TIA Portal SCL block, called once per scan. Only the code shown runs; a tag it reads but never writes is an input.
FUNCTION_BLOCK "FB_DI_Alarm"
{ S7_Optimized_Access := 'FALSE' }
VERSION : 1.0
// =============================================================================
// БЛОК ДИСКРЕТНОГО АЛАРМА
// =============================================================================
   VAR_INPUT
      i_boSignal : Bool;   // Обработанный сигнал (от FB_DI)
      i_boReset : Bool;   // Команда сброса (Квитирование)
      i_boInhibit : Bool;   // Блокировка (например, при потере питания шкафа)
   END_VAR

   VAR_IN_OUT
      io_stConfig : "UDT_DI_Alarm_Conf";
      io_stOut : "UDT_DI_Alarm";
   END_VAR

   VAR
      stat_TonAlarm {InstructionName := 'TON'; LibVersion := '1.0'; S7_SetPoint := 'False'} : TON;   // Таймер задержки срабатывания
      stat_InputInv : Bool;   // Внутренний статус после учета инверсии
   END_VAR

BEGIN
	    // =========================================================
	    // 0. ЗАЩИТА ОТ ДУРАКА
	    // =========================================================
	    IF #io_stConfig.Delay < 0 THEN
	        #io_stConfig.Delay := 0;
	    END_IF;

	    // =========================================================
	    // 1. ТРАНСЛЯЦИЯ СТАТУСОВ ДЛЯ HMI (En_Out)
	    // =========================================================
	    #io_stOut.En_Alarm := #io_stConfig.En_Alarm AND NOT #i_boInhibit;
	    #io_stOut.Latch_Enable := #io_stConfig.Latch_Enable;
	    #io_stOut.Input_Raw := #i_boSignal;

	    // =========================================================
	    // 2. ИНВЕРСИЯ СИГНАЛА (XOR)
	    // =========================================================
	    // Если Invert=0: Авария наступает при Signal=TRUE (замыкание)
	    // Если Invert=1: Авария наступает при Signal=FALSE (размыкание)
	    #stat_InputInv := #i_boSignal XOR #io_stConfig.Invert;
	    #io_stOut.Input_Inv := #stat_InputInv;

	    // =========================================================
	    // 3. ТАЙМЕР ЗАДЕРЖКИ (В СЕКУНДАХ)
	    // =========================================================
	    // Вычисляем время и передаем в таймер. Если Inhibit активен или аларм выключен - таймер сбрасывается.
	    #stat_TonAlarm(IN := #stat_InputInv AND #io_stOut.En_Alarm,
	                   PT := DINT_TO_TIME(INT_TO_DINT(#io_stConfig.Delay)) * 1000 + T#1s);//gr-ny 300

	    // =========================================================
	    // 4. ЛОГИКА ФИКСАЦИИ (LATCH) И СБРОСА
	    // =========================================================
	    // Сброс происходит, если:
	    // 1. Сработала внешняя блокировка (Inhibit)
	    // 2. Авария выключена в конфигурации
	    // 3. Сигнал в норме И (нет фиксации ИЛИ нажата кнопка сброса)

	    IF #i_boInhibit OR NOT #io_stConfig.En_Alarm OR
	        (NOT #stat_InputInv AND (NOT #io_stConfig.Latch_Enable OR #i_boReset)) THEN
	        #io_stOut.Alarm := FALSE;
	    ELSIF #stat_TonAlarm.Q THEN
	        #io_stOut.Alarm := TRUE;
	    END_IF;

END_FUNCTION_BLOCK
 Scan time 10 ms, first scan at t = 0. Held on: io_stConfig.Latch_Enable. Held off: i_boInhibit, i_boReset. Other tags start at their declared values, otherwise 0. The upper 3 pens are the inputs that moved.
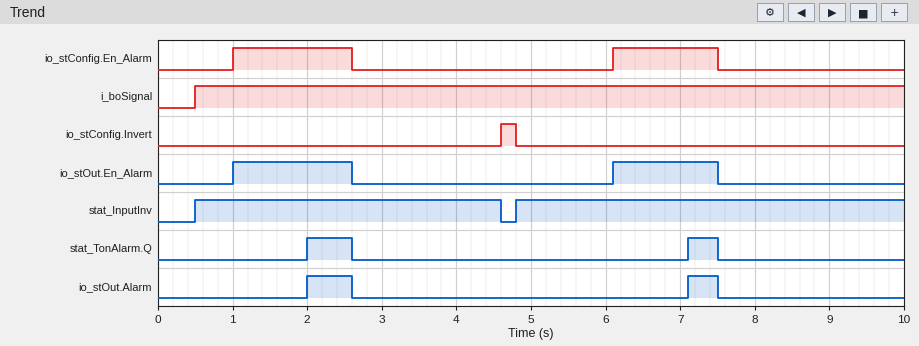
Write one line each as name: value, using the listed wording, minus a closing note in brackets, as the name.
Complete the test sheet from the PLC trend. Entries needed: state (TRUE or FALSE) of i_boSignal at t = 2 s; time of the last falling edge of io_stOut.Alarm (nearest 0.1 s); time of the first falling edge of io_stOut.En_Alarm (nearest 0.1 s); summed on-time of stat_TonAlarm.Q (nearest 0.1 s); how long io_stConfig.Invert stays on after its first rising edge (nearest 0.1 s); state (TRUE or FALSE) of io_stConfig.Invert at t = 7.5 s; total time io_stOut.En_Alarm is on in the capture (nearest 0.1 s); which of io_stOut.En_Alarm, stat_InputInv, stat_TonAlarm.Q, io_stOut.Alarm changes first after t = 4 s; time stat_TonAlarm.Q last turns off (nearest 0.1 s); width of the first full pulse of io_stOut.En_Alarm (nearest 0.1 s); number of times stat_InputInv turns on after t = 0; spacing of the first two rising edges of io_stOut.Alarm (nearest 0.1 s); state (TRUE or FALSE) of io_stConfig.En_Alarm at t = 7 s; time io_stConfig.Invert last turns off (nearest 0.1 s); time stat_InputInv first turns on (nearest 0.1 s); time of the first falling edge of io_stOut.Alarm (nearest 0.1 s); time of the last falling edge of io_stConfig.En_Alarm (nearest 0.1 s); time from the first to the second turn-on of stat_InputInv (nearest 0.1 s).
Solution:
state (TRUE or FALSE) of i_boSignal at t = 2 s: TRUE
time of the last falling edge of io_stOut.Alarm: 7.5 s
time of the first falling edge of io_stOut.En_Alarm: 2.6 s
summed on-time of stat_TonAlarm.Q: 1.0 s
how long io_stConfig.Invert stays on after its first rising edge: 0.2 s
state (TRUE or FALSE) of io_stConfig.Invert at t = 7.5 s: FALSE
total time io_stOut.En_Alarm is on in the capture: 3.0 s
which of io_stOut.En_Alarm, stat_InputInv, stat_TonAlarm.Q, io_stOut.Alarm changes first after t = 4 s: stat_InputInv
time stat_TonAlarm.Q last turns off: 7.5 s
width of the first full pulse of io_stOut.En_Alarm: 1.6 s
number of times stat_InputInv turns on after t = 0: 2
spacing of the first two rising edges of io_stOut.Alarm: 5.1 s
state (TRUE or FALSE) of io_stConfig.En_Alarm at t = 7 s: TRUE
time io_stConfig.Invert last turns off: 4.8 s
time stat_InputInv first turns on: 0.5 s
time of the first falling edge of io_stOut.Alarm: 2.6 s
time of the last falling edge of io_stConfig.En_Alarm: 7.5 s
time from the first to the second turn-on of stat_InputInv: 4.3 s
